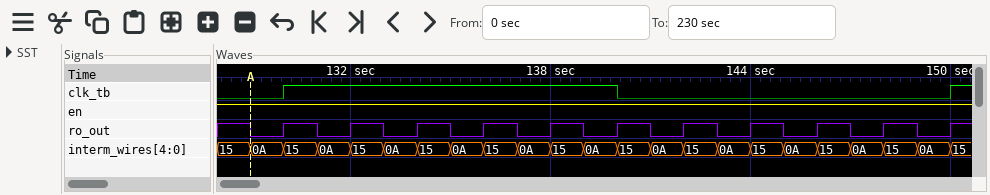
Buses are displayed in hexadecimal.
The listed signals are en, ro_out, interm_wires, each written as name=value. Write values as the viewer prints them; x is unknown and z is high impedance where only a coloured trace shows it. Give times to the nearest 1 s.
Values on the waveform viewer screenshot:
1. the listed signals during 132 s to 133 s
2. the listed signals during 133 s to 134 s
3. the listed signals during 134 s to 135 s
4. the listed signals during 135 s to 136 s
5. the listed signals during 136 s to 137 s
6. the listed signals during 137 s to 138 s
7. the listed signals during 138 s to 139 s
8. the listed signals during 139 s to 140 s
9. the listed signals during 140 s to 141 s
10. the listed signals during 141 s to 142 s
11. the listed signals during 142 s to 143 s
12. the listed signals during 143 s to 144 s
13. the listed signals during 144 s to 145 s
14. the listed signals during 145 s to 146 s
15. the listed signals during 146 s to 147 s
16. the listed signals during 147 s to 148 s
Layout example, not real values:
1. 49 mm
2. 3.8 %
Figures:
1. en=1, ro_out=1, interm_wires=15
2. en=1, ro_out=0, interm_wires=0A
3. en=1, ro_out=1, interm_wires=15
4. en=1, ro_out=0, interm_wires=0A
5. en=1, ro_out=1, interm_wires=15
6. en=1, ro_out=0, interm_wires=0A
7. en=1, ro_out=1, interm_wires=15
8. en=1, ro_out=0, interm_wires=0A
9. en=1, ro_out=1, interm_wires=15
10. en=1, ro_out=0, interm_wires=0A
11. en=1, ro_out=1, interm_wires=15
12. en=1, ro_out=0, interm_wires=0A
13. en=1, ro_out=1, interm_wires=15
14. en=1, ro_out=0, interm_wires=0A
15. en=1, ro_out=1, interm_wires=15
16. en=1, ro_out=0, interm_wires=0A
